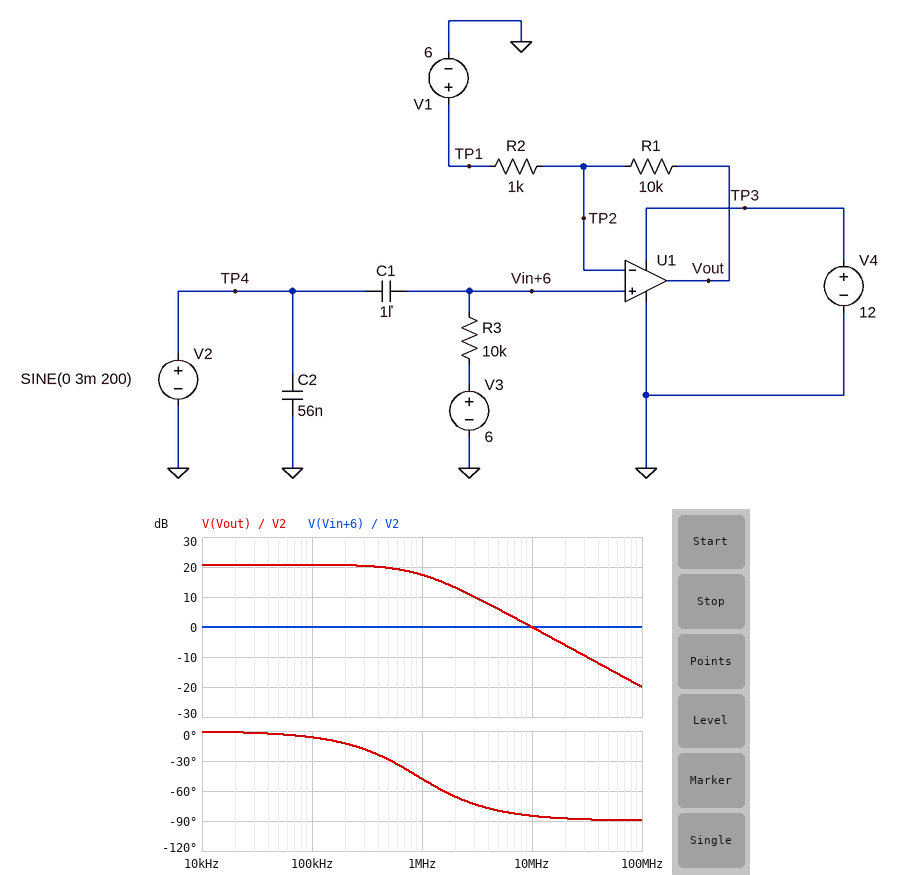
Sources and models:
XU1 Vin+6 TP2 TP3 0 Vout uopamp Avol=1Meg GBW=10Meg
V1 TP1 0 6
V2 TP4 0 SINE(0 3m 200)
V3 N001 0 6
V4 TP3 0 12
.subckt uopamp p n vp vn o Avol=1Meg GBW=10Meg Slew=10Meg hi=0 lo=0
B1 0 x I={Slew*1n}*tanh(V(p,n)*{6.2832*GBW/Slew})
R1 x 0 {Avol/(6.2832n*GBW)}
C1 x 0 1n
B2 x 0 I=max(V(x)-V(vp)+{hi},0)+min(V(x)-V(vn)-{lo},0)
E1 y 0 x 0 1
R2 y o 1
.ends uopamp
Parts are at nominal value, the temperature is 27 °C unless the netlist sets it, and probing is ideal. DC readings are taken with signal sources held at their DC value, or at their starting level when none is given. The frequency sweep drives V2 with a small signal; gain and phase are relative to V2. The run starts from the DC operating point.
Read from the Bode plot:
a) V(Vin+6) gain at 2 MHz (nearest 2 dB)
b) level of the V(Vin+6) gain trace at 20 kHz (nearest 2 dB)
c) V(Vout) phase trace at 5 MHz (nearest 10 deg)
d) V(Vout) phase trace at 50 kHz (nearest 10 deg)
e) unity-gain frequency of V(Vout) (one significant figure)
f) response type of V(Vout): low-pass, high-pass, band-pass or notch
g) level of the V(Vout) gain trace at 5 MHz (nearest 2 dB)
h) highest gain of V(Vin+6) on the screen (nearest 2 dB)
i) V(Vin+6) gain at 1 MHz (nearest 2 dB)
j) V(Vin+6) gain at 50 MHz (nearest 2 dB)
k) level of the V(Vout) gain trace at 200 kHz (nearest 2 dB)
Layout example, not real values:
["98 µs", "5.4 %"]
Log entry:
["0 dB", "0 dB", "-80 deg", "0 deg", "10 MHz", "low-pass", "6 dB", "0 dB", "0 dB", "0 dB", "20 dB"]
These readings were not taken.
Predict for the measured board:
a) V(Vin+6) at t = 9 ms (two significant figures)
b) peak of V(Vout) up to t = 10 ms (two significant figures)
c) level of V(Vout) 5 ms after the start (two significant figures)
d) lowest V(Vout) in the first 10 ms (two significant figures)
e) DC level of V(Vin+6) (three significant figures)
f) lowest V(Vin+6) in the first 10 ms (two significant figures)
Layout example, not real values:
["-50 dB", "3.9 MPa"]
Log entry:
["6.0 V", "6.0 V", "6.0 V", "6.0 V", "6.00 V", "6.0 V"]
